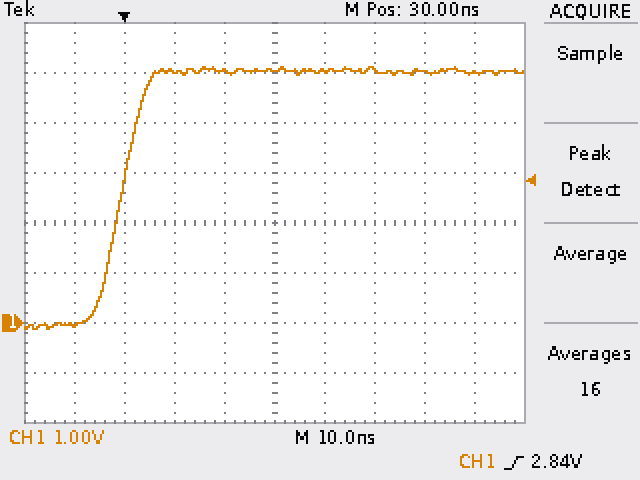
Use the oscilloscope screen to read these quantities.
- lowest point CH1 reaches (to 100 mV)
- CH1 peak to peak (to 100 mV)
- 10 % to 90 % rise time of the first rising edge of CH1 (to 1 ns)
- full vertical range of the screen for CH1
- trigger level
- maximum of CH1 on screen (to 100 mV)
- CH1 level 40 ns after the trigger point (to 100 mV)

-100 mV
5.2 V
9 ns
8 V
2.84 V
5.1 V
5.0 V
